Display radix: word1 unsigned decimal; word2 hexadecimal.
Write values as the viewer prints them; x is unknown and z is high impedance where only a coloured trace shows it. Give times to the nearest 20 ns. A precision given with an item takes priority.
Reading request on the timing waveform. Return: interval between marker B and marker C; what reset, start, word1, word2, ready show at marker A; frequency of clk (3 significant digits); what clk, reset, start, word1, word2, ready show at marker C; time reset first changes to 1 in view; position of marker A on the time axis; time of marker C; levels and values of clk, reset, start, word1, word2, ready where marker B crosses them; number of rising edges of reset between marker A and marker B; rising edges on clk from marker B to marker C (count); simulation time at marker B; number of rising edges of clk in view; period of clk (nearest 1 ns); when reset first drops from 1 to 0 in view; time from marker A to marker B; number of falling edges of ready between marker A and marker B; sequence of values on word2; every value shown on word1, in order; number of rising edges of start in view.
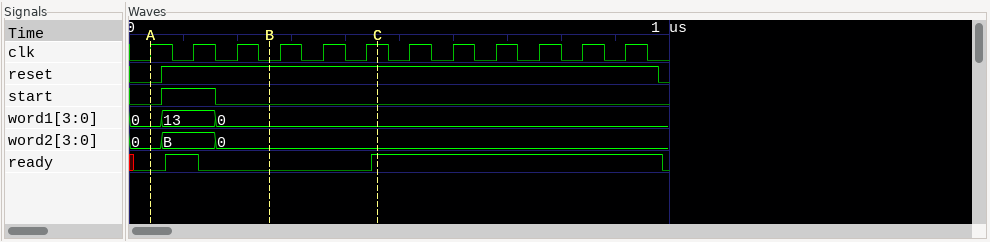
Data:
200 ns
reset=0, start=0, word1=0, word2=0, ready=0
12.5 MHz
clk=1, reset=1, start=0, word1=0, word2=0, ready=1
60 ns
40 ns
460 ns
clk=0, reset=1, start=0, word1=0, word2=0, ready=0
1
3
260 ns
12
80 ns
980 ns
220 ns
1
0, B, 0
0, 13, 0
1
